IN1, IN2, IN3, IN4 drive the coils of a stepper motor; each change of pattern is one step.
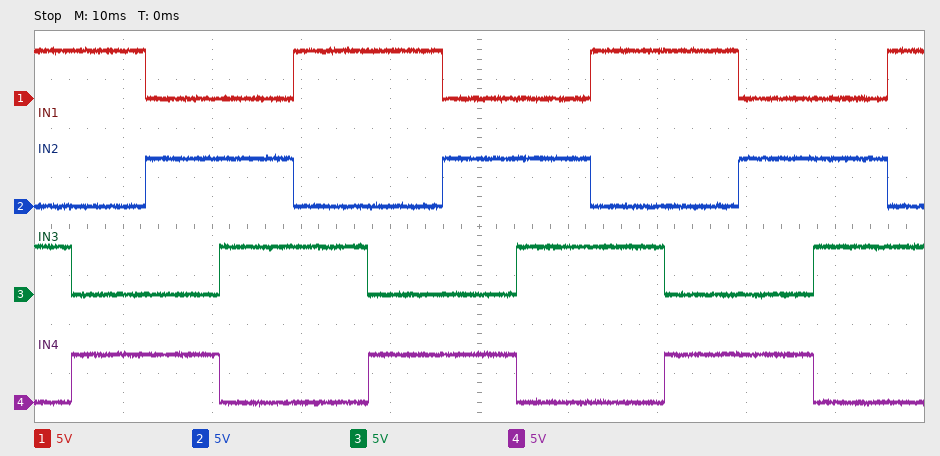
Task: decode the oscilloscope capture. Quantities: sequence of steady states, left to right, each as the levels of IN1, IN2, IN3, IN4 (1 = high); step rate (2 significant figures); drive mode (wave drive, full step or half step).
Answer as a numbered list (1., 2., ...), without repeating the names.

1. 1010 1001 0101 0110 1010 1001 0101 0110 1010 1001 0101 0110 1010
2. 120 steps/s
3. full step
